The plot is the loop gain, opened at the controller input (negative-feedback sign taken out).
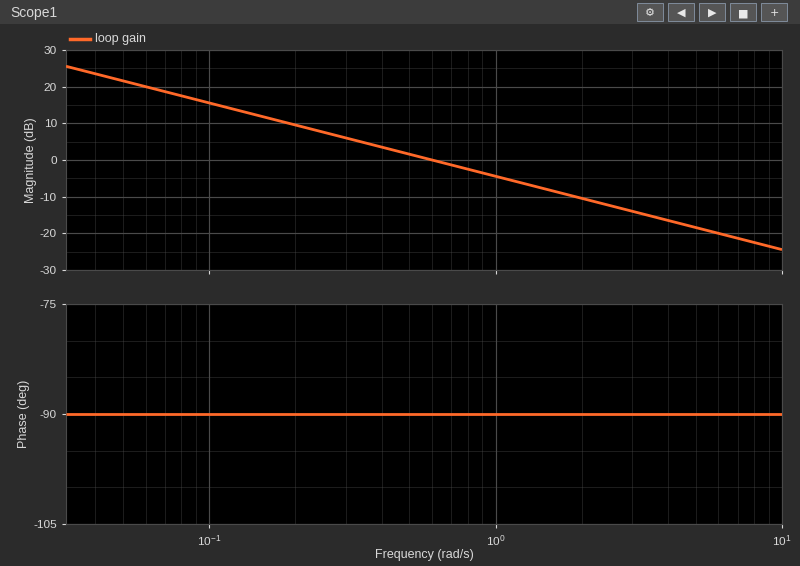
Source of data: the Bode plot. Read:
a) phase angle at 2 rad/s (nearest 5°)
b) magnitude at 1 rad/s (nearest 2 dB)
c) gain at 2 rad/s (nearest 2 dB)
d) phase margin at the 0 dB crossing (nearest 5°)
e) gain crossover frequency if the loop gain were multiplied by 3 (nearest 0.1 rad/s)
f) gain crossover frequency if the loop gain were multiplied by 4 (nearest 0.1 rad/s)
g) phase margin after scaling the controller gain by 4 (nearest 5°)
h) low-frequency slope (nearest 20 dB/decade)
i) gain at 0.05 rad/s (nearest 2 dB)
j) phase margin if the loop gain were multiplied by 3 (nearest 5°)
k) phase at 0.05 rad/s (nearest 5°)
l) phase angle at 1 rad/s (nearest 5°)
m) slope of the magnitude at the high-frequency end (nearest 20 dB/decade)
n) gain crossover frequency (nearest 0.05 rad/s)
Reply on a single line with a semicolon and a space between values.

-90°; -4 dB; -10 dB; 90°; 1.8 rad/s; 2.4 rad/s; 90°; -20 dB/decade; 22 dB; 90°; -90°; -90°; -20 dB/decade; 0.60 rad/s
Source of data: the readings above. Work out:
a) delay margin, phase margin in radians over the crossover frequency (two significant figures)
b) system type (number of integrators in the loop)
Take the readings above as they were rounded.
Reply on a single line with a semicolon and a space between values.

2.6 s; 1
